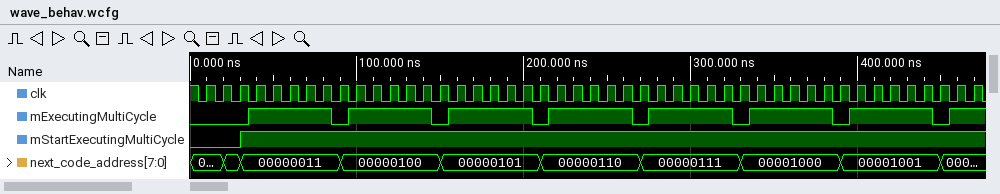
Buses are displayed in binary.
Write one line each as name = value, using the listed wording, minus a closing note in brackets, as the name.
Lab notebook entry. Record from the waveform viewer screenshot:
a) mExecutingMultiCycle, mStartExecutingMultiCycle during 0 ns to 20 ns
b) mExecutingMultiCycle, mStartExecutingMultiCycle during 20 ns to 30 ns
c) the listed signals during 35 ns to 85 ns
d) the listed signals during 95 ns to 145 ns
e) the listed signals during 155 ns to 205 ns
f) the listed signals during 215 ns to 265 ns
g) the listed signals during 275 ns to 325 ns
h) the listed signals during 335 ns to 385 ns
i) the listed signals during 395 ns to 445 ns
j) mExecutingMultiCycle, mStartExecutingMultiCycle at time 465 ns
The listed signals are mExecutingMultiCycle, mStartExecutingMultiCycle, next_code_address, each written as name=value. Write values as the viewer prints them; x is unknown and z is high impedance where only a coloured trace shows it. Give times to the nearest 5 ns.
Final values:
mExecutingMultiCycle, mStartExecutingMultiCycle during 0 ns to 20 ns = mExecutingMultiCycle=0, mStartExecutingMultiCycle=0
mExecutingMultiCycle, mStartExecutingMultiCycle during 20 ns to 30 ns = mExecutingMultiCycle=0, mStartExecutingMultiCycle=0
the listed signals during 35 ns to 85 ns = mExecutingMultiCycle=1, mStartExecutingMultiCycle=1, next_code_address=00000011
the listed signals during 95 ns to 145 ns = mExecutingMultiCycle=1, mStartExecutingMultiCycle=1, next_code_address=00000100
the listed signals during 155 ns to 205 ns = mExecutingMultiCycle=1, mStartExecutingMultiCycle=1, next_code_address=00000101
the listed signals during 215 ns to 265 ns = mExecutingMultiCycle=1, mStartExecutingMultiCycle=1, next_code_address=00000110
the listed signals during 275 ns to 325 ns = mExecutingMultiCycle=1, mStartExecutingMultiCycle=1, next_code_address=00000111
the listed signals during 335 ns to 385 ns = mExecutingMultiCycle=1, mStartExecutingMultiCycle=1, next_code_address=00001000
the listed signals during 395 ns to 445 ns = mExecutingMultiCycle=1, mStartExecutingMultiCycle=1, next_code_address=00001001
mExecutingMultiCycle, mStartExecutingMultiCycle at time 465 ns = mExecutingMultiCycle=1, mStartExecutingMultiCycle=1
